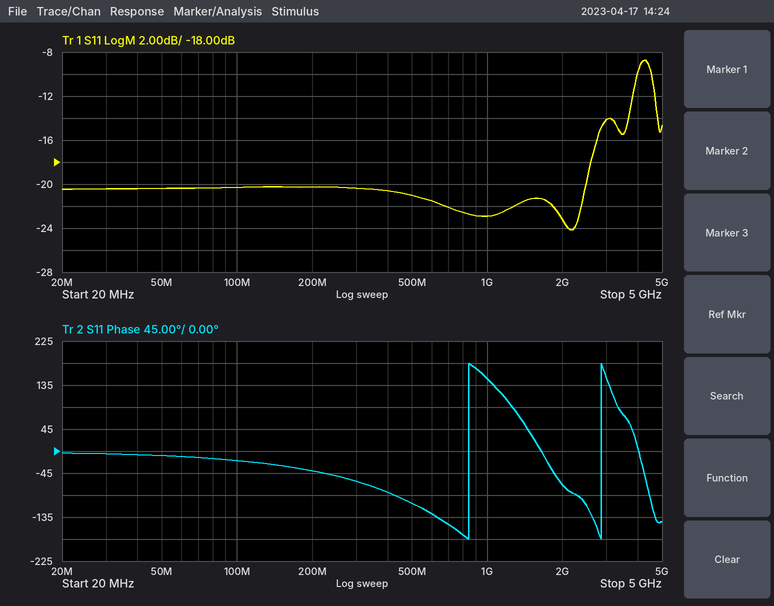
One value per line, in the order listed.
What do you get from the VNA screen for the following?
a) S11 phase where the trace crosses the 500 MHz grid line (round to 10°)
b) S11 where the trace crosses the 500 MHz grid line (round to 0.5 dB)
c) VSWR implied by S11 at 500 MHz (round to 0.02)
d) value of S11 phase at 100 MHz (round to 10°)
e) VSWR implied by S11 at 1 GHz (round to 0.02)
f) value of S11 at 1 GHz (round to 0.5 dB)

-110°
-21.0 dB
1.20
-20°
1.16
-23.0 dB
